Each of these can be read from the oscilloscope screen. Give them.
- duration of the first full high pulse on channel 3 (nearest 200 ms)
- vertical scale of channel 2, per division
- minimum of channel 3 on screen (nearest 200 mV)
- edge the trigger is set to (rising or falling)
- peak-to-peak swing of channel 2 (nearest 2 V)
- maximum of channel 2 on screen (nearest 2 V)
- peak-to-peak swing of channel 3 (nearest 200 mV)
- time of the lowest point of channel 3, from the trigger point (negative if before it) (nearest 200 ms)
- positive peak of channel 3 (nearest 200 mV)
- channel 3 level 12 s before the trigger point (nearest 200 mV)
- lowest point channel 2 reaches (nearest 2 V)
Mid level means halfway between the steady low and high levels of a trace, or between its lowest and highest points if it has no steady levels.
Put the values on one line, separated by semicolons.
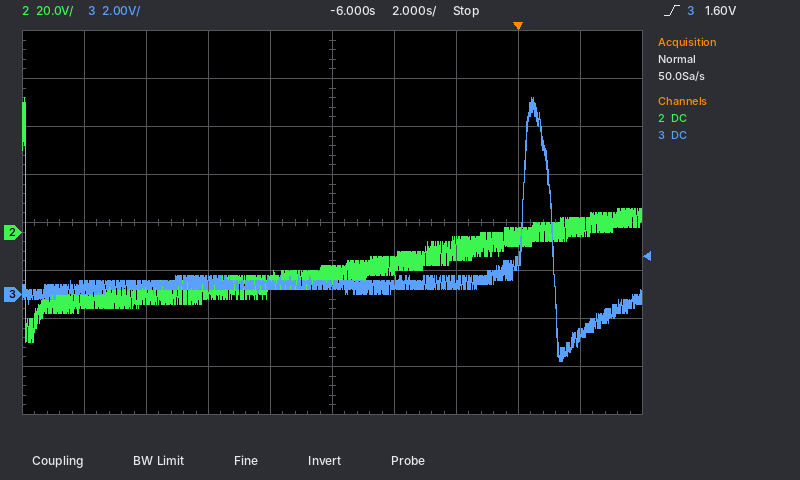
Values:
1.0 s; 20 V; -2.8 V; rising; 102 V; 56 V; 11.0 V; +1.4 s; 8.2 V; 400 mV; -46 V
